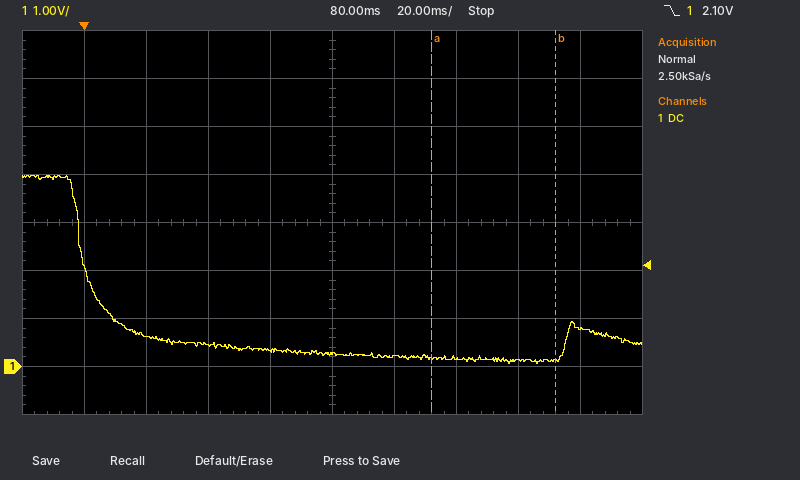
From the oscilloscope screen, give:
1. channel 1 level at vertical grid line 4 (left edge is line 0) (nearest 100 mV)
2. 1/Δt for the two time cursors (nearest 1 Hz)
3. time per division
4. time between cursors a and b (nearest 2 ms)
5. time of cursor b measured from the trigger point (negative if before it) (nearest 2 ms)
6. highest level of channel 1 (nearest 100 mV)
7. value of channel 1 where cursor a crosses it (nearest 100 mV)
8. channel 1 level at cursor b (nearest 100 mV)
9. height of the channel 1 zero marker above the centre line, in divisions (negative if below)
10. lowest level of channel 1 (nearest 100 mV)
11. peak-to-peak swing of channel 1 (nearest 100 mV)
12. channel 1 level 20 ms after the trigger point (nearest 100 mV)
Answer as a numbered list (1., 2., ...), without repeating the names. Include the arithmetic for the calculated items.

1. 300 mV
2. 1 / 40 ms ≈ 25 Hz
3. 20 ms
4. 40 ms
5. +152 ms
6. 4.0 V
7. 200 mV
8. 100 mV
9. -3.0 div
10. 100 mV
11. 4.0 V − (100 mV) = 3.9 V
12. 600 mV
